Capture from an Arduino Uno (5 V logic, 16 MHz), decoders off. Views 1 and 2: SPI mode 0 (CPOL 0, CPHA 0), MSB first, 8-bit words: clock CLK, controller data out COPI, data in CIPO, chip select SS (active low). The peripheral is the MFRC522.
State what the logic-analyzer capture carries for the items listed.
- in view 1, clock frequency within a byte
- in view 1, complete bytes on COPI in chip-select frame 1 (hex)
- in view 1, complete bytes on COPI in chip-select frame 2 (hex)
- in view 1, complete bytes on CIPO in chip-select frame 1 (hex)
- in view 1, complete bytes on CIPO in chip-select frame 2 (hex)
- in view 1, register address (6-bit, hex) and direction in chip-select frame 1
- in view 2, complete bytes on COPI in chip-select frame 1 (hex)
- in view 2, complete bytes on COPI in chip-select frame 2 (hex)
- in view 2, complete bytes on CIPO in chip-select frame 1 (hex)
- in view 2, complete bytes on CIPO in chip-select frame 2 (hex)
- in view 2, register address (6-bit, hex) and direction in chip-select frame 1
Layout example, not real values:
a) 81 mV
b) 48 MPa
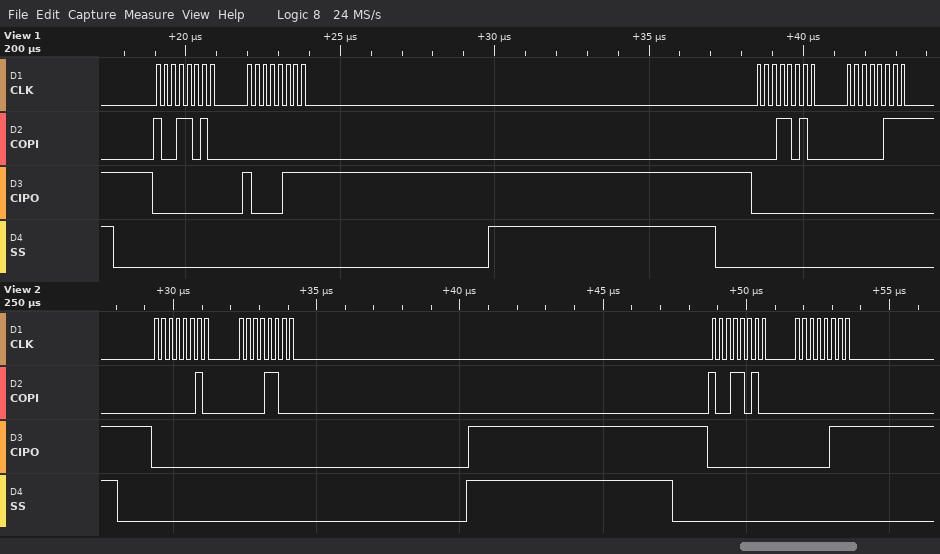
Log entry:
a) 4 MHz
b) 0x9A 0x00
c) 0x1A 0x07
d) 0x00 0x87
e) 0x00 0x00
f) 0x0D read
g) 02 0C
h) 9A 00
i) 00 00
j) 00 07
k) 0x01 write
